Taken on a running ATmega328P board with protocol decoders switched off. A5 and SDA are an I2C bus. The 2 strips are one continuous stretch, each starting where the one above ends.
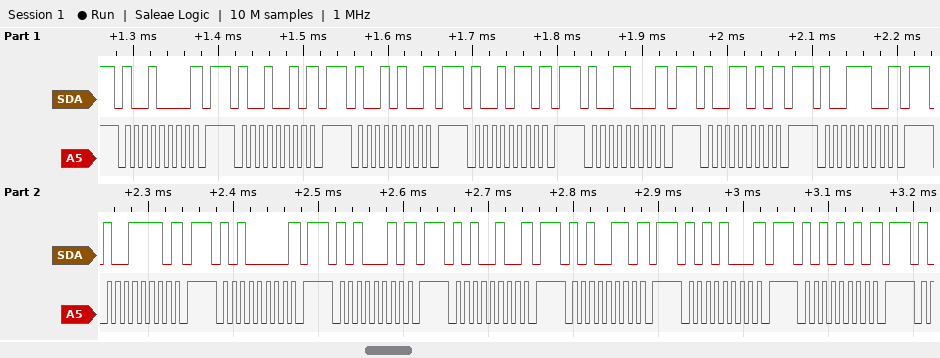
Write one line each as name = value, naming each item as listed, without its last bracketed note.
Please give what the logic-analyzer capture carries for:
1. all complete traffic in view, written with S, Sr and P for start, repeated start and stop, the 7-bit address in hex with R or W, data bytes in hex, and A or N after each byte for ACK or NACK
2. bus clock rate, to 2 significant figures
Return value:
all complete traffic in view, written with S, Sr and P for start, repeated start and stop, the 7-bit address in hex with R or W, data bytes in hex, and A or N after each byte for ACK or NACK = S 48W N P S 49W N P S 4AW N P S 4BW N P S 4CW N P S 4DW N P S 4EW N P S 4FW N P S 50W N P S 51W N P S 52W N P S 53W N P S 54W N P S 55W N P
bus clock rate, to 2 significant figures = 100 kHz
